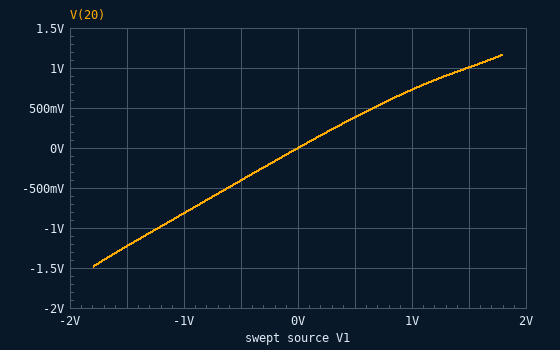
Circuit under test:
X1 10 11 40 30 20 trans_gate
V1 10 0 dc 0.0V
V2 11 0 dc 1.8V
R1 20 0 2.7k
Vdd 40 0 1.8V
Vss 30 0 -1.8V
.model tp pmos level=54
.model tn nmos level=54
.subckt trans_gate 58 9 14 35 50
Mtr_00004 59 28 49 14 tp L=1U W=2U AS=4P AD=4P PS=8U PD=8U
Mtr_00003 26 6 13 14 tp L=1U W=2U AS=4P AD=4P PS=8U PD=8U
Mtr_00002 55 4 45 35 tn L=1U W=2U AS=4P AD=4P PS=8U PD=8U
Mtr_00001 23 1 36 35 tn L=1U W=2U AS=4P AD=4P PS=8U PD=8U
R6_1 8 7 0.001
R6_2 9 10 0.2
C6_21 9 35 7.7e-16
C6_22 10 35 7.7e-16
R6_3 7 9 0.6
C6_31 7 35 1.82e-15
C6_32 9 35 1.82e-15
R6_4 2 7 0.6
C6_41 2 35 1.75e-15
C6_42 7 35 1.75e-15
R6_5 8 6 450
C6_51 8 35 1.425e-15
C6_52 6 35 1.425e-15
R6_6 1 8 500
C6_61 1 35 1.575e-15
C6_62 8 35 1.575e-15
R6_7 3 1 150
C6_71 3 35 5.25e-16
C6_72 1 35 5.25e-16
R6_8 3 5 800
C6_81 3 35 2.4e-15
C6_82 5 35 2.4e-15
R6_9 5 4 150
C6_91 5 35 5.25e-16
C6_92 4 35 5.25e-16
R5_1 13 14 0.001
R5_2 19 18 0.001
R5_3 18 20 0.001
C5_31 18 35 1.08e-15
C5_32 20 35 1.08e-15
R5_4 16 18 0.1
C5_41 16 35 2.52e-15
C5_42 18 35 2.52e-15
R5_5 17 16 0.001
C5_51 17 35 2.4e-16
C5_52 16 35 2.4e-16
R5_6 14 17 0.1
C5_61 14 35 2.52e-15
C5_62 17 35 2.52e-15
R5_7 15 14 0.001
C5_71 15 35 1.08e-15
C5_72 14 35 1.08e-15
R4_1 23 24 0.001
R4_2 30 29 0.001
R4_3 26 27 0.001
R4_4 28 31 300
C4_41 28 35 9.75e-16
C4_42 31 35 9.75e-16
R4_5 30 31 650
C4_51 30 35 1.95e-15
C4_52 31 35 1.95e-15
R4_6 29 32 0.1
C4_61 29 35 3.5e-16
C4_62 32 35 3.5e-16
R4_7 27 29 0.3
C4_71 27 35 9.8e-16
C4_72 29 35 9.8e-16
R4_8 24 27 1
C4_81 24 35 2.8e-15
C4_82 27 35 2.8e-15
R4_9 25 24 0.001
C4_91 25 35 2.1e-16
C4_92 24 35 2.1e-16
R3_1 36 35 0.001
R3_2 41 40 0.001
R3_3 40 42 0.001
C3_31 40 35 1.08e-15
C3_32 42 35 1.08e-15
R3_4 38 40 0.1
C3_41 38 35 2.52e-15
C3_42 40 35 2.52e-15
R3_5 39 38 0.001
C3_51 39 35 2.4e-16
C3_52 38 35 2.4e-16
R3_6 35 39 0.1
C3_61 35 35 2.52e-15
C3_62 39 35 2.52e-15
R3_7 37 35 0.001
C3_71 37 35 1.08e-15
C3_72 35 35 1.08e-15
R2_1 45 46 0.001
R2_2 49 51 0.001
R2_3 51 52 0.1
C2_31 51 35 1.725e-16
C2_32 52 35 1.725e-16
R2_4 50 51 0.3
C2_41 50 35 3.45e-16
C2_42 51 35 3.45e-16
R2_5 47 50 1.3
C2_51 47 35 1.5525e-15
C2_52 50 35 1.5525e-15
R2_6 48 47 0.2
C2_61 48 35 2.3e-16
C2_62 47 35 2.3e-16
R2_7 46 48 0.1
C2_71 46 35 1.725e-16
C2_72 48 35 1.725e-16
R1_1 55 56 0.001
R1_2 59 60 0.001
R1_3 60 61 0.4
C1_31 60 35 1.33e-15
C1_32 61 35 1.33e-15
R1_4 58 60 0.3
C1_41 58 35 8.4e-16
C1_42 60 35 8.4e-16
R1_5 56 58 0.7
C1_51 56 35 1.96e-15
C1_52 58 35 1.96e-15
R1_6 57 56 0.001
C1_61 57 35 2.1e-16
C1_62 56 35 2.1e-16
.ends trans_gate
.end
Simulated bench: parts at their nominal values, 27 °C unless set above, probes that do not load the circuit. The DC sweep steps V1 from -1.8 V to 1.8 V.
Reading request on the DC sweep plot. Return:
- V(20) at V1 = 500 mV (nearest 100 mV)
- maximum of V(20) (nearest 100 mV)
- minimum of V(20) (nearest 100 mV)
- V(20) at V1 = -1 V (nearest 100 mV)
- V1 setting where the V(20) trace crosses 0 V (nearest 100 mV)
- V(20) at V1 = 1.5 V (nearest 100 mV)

400 mV
1.2 V
-1.5 V
-800 mV
0 V
1.0 V
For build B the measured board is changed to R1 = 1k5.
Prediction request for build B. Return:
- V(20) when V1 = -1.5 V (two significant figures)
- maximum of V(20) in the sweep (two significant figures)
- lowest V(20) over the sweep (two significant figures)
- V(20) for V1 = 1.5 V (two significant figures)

-1.1 V
940 mV
-1.3 V
820 mV
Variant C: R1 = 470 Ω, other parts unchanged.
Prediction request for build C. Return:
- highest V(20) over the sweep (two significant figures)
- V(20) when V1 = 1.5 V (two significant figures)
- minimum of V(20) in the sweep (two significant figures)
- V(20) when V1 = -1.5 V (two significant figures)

490 mV
430 mV
-730 mV
-610 mV
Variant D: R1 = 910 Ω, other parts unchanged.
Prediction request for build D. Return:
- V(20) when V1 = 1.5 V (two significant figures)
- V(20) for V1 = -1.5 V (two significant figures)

650 mV
-870 mV
